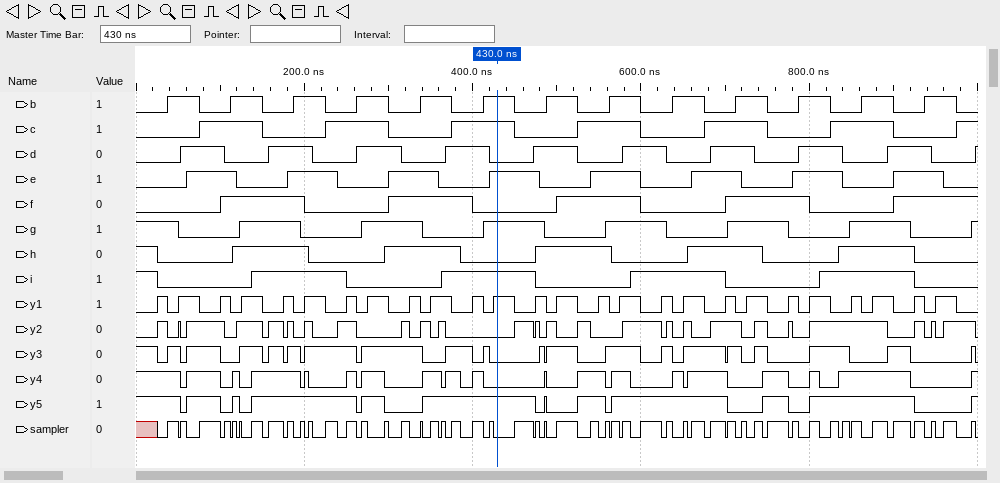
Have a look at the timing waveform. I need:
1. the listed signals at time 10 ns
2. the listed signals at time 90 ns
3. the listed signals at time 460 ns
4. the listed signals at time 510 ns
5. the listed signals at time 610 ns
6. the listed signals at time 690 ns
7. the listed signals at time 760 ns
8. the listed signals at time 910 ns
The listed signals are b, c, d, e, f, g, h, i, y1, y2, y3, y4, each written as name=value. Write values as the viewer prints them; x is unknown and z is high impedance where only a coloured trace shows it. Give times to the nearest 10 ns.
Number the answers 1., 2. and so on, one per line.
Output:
1. b=0, c=0, d=0, e=0, f=0, g=1, h=1, i=1, y1=0, y2=0, y3=1, y4=1
2. b=0, c=1, d=1, e=1, f=0, g=0, h=0, i=0, y1=0, y2=1, y3=1, y4=1
3. b=0, c=0, d=0, e=1, f=0, g=1, h=0, i=1, y1=0, y2=1, y3=0, y4=0
4. b=1, c=0, d=1, e=0, f=1, g=0, h=1, i=0, y1=1, y2=0, y3=1, y4=0
5. b=0, c=0, d=1, e=0, f=0, g=1, h=0, i=1, y1=0, y2=1, y3=0, y4=0
6. b=0, c=1, d=1, e=1, f=0, g=0, h=1, i=1, y1=0, y2=1, y3=1, y4=1
7. b=0, c=0, d=0, e=0, f=1, g=1, h=0, i=0, y1=0, y2=0, y3=0, y4=1
8. b=0, c=0, d=1, e=1, f=1, g=1, h=1, i=1, y1=0, y2=0, y3=1, y4=1
